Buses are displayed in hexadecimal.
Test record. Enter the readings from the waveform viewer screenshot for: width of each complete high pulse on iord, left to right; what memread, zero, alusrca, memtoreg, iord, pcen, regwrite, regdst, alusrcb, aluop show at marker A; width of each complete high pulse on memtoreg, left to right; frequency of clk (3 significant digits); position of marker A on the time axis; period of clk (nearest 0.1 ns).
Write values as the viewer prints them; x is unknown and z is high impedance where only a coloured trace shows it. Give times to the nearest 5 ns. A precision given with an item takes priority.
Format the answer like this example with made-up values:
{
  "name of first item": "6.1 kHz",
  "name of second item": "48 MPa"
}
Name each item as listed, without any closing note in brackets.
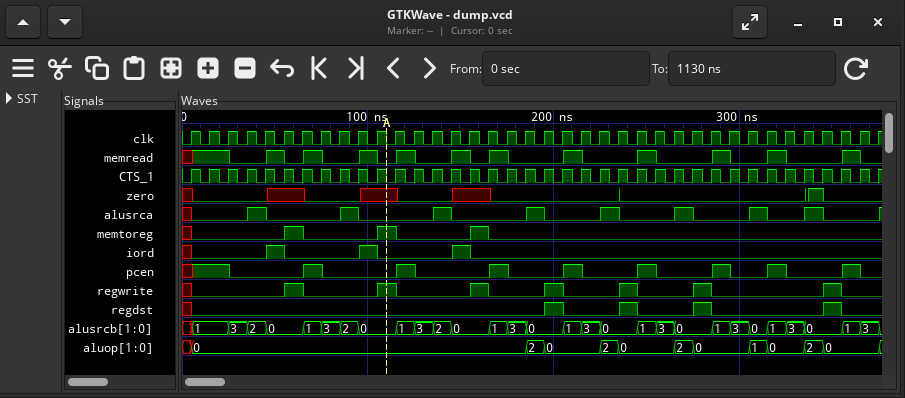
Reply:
{
  "width of each complete high pulse on iord, left to right": "10 ns, 10 ns, 10 ns",
  "what memread, zero, alusrca, memtoreg, iord, pcen, regwrite, regdst, alusrcb, aluop show at marker A": "memread=0, zero=x, alusrca=0, memtoreg=1, iord=0, pcen=0, regwrite=1, regdst=0, alusrcb=0, aluop=0",
  "width of each complete high pulse on memtoreg, left to right": "10 ns, 10 ns, 10 ns",
  "frequency of clk": "100 MHz",
  "position of marker A on the time axis": "110 ns",
  "period of clk": "10 ns"
}
